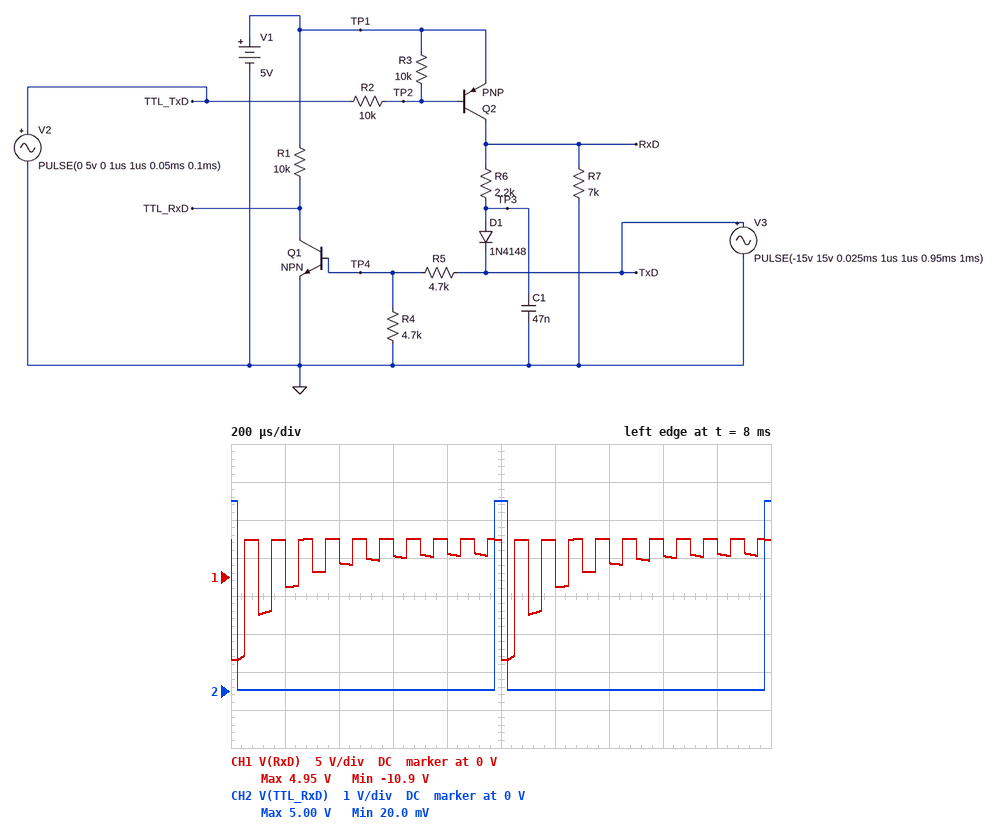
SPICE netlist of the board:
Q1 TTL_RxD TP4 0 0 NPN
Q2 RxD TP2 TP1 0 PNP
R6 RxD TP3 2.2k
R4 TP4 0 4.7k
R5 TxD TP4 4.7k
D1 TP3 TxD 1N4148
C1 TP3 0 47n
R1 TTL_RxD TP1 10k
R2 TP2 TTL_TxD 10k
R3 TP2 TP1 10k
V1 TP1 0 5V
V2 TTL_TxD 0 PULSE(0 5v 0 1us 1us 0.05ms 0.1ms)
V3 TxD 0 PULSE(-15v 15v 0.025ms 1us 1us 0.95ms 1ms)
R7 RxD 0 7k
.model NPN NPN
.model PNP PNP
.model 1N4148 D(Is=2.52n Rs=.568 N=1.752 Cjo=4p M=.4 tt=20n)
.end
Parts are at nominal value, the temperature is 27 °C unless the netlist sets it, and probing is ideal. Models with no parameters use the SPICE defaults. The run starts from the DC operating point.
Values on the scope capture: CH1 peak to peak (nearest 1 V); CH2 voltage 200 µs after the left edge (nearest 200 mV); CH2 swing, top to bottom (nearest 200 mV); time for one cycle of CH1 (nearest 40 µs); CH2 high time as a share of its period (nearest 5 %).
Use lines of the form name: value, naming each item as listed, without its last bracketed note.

CH1 peak to peak: 16 V
CH2 voltage 200 µs after the left edge: 0 V
CH2 swing, top to bottom: 5.0 V
time for one cycle of CH1: 1.00 ms
CH2 high time as a share of its period: 5 %
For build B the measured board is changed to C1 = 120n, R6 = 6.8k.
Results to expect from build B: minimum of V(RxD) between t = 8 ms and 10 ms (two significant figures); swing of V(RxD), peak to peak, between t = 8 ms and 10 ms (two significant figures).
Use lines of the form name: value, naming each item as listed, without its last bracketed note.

minimum of V(RxD) between t = 8 ms and 10 ms: -7.3 V
swing of V(RxD), peak to peak, between t = 8 ms and 10 ms: 12 V
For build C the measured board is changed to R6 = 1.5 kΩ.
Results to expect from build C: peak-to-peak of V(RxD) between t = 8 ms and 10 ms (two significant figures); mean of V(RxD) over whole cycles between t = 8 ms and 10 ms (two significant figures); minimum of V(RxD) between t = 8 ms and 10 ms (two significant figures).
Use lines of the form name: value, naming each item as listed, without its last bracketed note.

peak-to-peak of V(RxD) between t = 8 ms and 10 ms: 17 V
mean of V(RxD) over whole cycles between t = 8 ms and 10 ms: 2.8 V
minimum of V(RxD) between t = 8 ms and 10 ms: -12 V
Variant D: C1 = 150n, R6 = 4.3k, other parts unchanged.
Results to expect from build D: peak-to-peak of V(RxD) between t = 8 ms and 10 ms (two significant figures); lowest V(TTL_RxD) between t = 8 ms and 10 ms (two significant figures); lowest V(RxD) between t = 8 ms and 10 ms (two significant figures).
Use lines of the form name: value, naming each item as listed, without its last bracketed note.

peak-to-peak of V(RxD) between t = 8 ms and 10 ms: 14 V
lowest V(TTL_RxD) between t = 8 ms and 10 ms: 20 mV
lowest V(RxD) between t = 8 ms and 10 ms: -8.9 V
